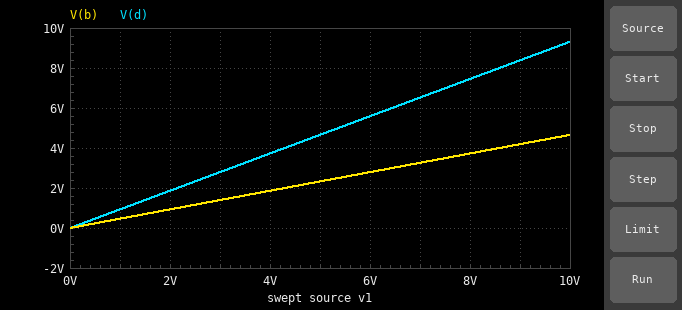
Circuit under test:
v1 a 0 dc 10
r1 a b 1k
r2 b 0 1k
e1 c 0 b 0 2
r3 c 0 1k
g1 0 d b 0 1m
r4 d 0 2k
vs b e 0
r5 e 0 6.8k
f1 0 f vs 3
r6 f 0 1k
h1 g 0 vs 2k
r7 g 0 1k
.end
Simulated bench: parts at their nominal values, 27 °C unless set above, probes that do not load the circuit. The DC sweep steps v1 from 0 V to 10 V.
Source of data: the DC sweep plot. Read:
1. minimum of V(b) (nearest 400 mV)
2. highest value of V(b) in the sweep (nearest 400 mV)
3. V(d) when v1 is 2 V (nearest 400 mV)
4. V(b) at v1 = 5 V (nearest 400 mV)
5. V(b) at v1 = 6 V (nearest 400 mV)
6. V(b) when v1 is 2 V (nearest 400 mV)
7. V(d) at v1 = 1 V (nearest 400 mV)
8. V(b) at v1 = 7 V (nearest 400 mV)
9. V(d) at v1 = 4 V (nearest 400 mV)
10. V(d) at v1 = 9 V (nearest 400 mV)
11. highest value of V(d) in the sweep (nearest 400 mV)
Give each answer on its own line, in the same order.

0 V
4.8 V
2.0 V
2.4 V
2.8 V
800 mV
800 mV
3.2 V
3.6 V
8.4 V
9.2 V
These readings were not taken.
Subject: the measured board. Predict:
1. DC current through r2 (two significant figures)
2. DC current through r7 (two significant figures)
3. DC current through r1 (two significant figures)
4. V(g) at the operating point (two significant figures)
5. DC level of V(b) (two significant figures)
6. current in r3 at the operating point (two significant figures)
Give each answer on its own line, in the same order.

4.7 mA
1.4 mA
5.3 mA
1.4 V
4.7 V
9.3 mA
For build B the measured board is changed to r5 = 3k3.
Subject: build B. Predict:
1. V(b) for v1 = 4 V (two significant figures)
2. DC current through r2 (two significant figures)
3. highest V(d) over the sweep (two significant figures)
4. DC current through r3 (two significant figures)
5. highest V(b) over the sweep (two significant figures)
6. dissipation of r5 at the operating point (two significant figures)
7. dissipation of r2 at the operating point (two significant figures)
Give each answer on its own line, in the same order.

1.7 V
4.3 mA
8.7 V
8.7 mA
4.3 V
5.7 mW
19 mW
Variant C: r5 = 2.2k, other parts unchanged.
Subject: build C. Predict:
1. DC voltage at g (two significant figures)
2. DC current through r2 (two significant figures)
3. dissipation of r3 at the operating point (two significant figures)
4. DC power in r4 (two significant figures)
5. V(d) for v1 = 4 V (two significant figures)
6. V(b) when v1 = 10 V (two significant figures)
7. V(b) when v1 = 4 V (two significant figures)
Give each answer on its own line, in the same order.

3.7 V
4.1 mA
66 mW
33 mW
3.3 V
4.1 V
1.6 V
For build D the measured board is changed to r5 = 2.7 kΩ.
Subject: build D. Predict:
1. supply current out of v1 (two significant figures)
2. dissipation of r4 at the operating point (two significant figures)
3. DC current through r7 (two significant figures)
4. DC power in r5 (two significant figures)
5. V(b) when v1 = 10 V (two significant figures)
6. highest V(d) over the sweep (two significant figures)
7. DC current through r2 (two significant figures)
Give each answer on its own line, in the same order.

5.8 mA
36 mW
3.1 mA
6.6 mW
4.2 V
8.4 V
4.2 mA
